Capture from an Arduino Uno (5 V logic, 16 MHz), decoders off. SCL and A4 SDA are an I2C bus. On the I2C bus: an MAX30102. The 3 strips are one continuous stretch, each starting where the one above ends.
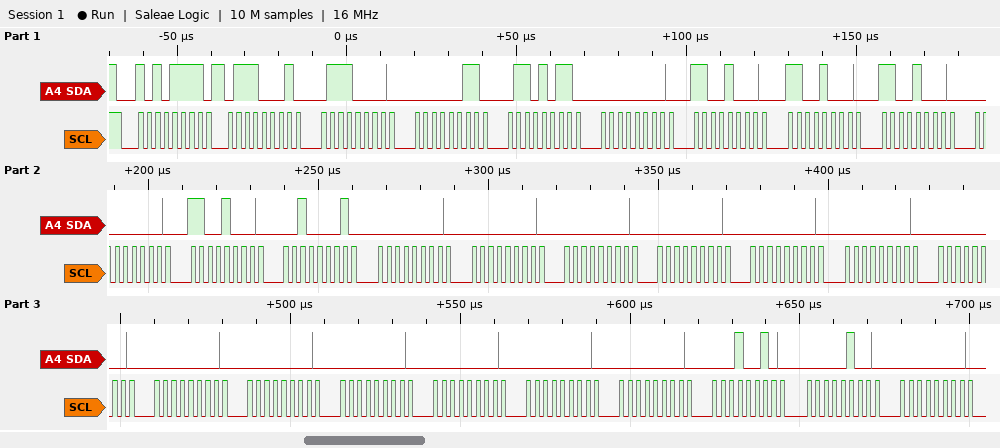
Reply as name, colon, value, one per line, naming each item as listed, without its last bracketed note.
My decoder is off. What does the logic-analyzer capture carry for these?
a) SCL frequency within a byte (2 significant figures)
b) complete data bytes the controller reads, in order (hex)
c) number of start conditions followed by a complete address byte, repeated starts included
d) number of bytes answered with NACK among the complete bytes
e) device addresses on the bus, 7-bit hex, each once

SCL frequency within a byte: 400 kHz
complete data bytes the controller reads, in order: 71 70 03 6B 00 C8 C8 C8 00 C8 21 00 00 00 00 00 00 00 00 00 00 00 00 00 12 04 00
number of start conditions followed by a complete address byte, repeated starts included: 1
number of bytes answered with NACK among the complete bytes: 0
device addresses on the bus, 7-bit hex, each once: 0x57
